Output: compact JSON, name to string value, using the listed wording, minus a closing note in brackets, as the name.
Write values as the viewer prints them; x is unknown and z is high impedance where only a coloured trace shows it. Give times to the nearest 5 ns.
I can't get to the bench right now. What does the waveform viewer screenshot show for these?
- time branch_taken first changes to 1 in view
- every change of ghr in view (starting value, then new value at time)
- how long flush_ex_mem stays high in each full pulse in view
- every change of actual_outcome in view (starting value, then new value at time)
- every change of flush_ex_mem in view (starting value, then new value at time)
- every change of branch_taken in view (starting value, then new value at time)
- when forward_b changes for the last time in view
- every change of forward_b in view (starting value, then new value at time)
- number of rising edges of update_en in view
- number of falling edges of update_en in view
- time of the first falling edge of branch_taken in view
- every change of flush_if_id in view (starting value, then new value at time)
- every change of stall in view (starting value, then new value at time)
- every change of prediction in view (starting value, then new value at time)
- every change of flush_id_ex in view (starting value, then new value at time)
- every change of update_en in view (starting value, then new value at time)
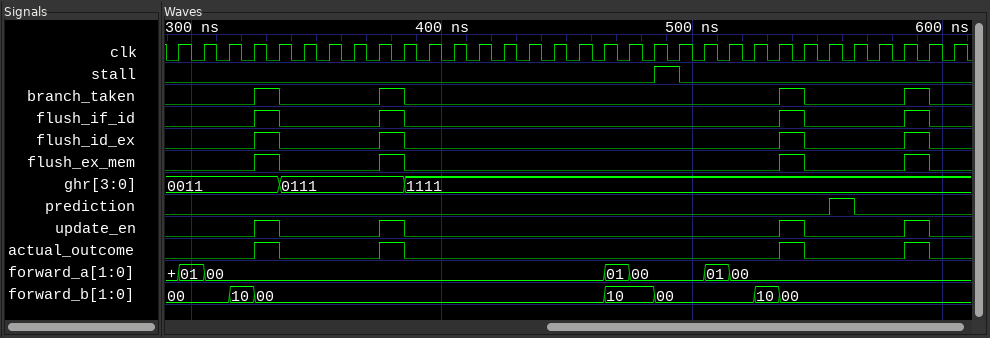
{"time branch_taken first changes to 1 in view": "325 ns", "every change of ghr in view": "0011, 0111 at 335 ns, 1111 at 385 ns", "how long flush_ex_mem stays high in each full pulse in view": "10 ns, 10 ns, 10 ns, 10 ns", "every change of actual_outcome in view": "0, 1 at 325 ns, 0 at 335 ns, 1 at 375 ns, 0 at 385 ns, 1 at 535 ns, 0 at 545 ns, 1 at 585 ns, 0 at 595 ns", "every change of flush_ex_mem in view": "0, 1 at 325 ns, 0 at 335 ns, 1 at 375 ns, 0 at 385 ns, 1 at 535 ns, 0 at 545 ns, 1 at 585 ns, 0 at 595 ns", "every change of branch_taken in view": "0, 1 at 325 ns, 0 at 335 ns, 1 at 375 ns, 0 at 385 ns, 1 at 535 ns, 0 at 545 ns, 1 at 585 ns, 0 at 595 ns", "when forward_b changes for the last time in view": "535 ns", "every change of forward_b in view": "00, 10 at 315 ns, 00 at 325 ns, 10 at 465 ns, 00 at 485 ns, 10 at 525 ns, 00 at 535 ns", "number of rising edges of update_en in view": "4", "number of falling edges of update_en in view": "4", "time of the first falling edge of branch_taken in view": "335 ns", "every change of flush_if_id in view": "0, 1 at 325 ns, 0 at 335 ns, 1 at 375 ns, 0 at 385 ns, 1 at 535 ns, 0 at 545 ns, 1 at 585 ns, 0 at 595 ns", "every change of stall in view": "0, 1 at 485 ns, 0 at 495 ns", "every change of prediction in view": "0, 1 at 555 ns, 0 at 565 ns", "every change of flush_id_ex in view": "0, 1 at 325 ns, 0 at 335 ns, 1 at 375 ns, 0 at 385 ns, 1 at 535 ns, 0 at 545 ns, 1 at 585 ns, 0 at 595 ns", "every change of update_en in view": "0, 1 at 325 ns, 0 at 335 ns, 1 at 375 ns, 0 at 385 ns, 1 at 535 ns, 0 at 545 ns, 1 at 585 ns, 0 at 595 ns"}
